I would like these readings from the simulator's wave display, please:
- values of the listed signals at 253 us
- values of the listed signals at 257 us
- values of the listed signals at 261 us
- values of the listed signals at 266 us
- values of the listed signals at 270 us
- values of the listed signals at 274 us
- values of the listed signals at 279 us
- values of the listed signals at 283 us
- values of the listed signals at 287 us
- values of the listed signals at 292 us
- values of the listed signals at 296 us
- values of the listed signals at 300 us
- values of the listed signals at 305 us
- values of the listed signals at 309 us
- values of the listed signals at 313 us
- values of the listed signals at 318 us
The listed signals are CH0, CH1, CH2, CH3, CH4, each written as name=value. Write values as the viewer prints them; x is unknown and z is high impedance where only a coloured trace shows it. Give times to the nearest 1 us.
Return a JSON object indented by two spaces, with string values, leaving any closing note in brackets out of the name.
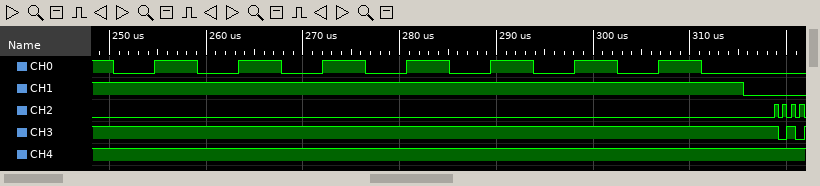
{
  "values of the listed signals at 253 us": "CH0=0, CH1=1, CH2=0, CH3=1, CH4=1",
  "values of the listed signals at 257 us": "CH0=1, CH1=1, CH2=0, CH3=1, CH4=1",
  "values of the listed signals at 261 us": "CH0=0, CH1=1, CH2=0, CH3=1, CH4=1",
  "values of the listed signals at 266 us": "CH0=1, CH1=1, CH2=0, CH3=1, CH4=1",
  "values of the listed signals at 270 us": "CH0=0, CH1=1, CH2=0, CH3=1, CH4=1",
  "values of the listed signals at 274 us": "CH0=1, CH1=1, CH2=0, CH3=1, CH4=1",
  "values of the listed signals at 279 us": "CH0=0, CH1=1, CH2=0, CH3=1, CH4=1",
  "values of the listed signals at 283 us": "CH0=1, CH1=1, CH2=0, CH3=1, CH4=1",
  "values of the listed signals at 287 us": "CH0=0, CH1=1, CH2=0, CH3=1, CH4=1",
  "values of the listed signals at 292 us": "CH0=1, CH1=1, CH2=0, CH3=1, CH4=1",
  "values of the listed signals at 296 us": "CH0=0, CH1=1, CH2=0, CH3=1, CH4=1",
  "values of the listed signals at 300 us": "CH0=1, CH1=1, CH2=0, CH3=1, CH4=1",
  "values of the listed signals at 305 us": "CH0=0, CH1=1, CH2=0, CH3=1, CH4=1",
  "values of the listed signals at 309 us": "CH0=1, CH1=1, CH2=0, CH3=1, CH4=1",
  "values of the listed signals at 313 us": "CH0=0, CH1=1, CH2=0, CH3=1, CH4=1",
  "values of the listed signals at 318 us": "CH0=0, CH1=0, CH2=0, CH3=1, CH4=1"
}
